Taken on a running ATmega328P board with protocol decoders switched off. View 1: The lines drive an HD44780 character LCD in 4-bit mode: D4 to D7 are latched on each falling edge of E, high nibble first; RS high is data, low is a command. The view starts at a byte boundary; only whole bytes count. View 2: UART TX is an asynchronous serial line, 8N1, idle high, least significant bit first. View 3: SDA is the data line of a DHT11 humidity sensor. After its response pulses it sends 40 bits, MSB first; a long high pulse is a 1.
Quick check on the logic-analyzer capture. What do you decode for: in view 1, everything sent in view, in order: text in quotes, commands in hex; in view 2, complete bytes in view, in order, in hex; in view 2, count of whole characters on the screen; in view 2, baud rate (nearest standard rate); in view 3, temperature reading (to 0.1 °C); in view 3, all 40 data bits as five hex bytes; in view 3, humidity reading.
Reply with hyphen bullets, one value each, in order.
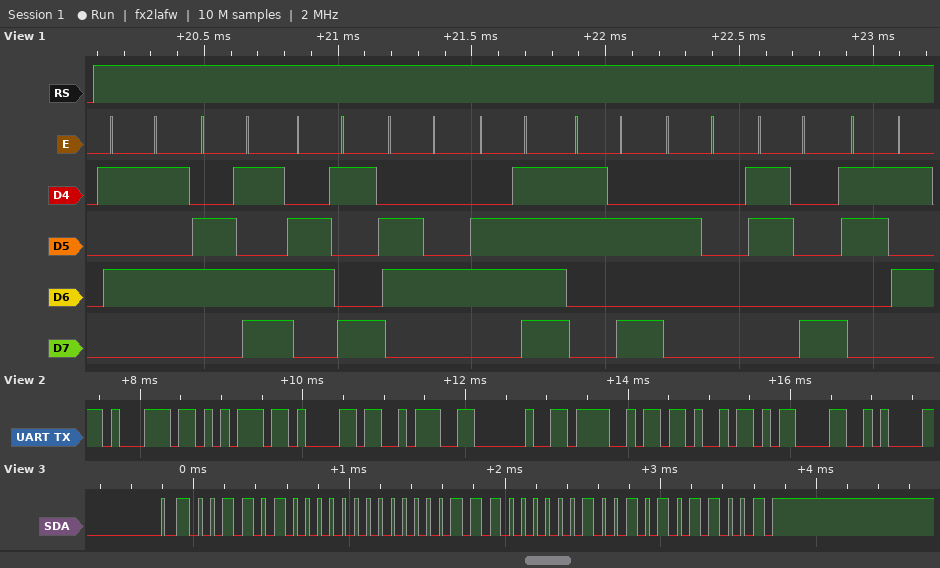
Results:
- "Umido: 85"
- 71 75 61 3A 20 4F 4B 0D 0A
- 9
- 9600 baud
- 28.9 °C
- 34 00 1C 09 59
- 52 %
